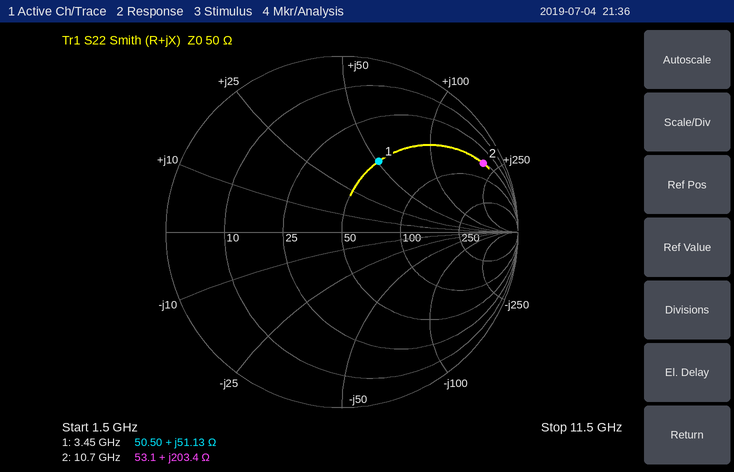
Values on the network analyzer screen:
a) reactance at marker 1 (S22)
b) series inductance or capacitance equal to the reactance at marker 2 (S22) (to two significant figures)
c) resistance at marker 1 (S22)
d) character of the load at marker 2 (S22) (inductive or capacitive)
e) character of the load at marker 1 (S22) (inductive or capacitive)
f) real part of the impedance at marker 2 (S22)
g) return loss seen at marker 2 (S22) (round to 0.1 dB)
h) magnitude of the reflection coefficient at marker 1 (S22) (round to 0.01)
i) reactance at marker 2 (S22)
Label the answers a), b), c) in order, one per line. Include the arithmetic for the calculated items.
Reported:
a) +51.13 Ω
b) L = 203.4 Ω/(2π × 10.7 GHz) ≈ 3.0 nH
c) 50.50 Ω
d) inductive
e) inductive
f) 53.1 Ω
g) 1.0 dB
h) 0.45
i) +203.4 Ω
